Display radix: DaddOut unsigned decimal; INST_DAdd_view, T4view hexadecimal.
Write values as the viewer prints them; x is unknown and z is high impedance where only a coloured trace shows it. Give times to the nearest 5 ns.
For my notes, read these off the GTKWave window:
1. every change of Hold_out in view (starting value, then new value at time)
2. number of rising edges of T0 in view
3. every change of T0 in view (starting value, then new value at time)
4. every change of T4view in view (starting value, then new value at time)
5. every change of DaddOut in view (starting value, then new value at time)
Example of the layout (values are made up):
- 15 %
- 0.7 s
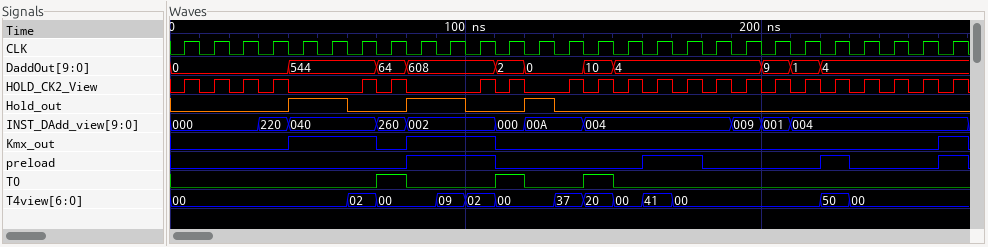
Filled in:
- 0, 1 at 40 ns, 0 at 60 ns, 1 at 80 ns, 0 at 100 ns, 1 at 120 ns, 0 at 130 ns
- 3
- 0, 1 at 70 ns, 0 at 80 ns, 1 at 110 ns, 0 at 120 ns, 1 at 140 ns, 0 at 150 ns
- 00, 02 at 60 ns, 00 at 70 ns, 09 at 90 ns, 02 at 100 ns, 00 at 110 ns, 37 at 130 ns, 20 at 140 ns, 00 at 150 ns, 41 at 160 ns, 00 at 170 ns, 50 at 220 ns, 00 at 230 ns
- 0, 544 at 40 ns, 64 at 70 ns, 608 at 80 ns, 2 at 110 ns, 0 at 120 ns, 10 at 140 ns, 4 at 150 ns, 9 at 200 ns, 1 at 210 ns, 4 at 220 ns
